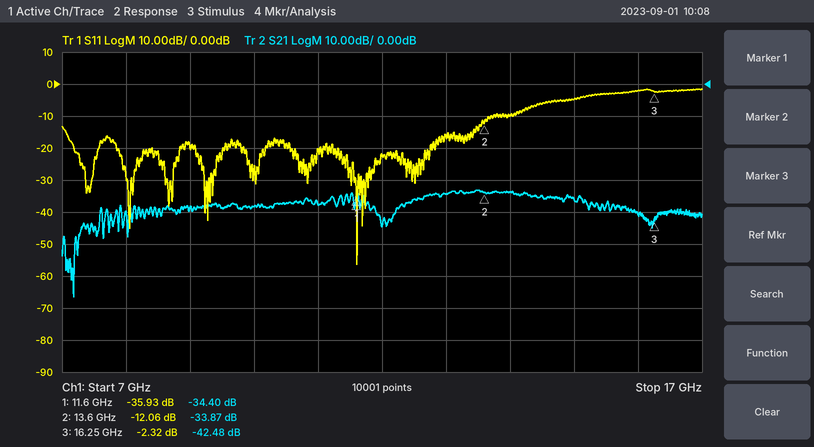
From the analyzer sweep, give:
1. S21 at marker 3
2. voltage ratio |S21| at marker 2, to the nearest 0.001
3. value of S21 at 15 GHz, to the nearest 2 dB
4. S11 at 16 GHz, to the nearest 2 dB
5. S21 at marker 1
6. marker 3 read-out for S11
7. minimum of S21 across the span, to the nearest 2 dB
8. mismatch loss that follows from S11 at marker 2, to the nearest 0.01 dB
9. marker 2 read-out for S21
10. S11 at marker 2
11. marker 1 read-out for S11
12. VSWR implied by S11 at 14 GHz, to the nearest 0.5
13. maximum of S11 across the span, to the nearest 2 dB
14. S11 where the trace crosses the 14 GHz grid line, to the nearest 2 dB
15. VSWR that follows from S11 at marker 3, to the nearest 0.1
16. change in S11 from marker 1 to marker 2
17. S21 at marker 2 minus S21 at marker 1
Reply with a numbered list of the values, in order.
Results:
1. -42.48 dB
2. 0.020
3. -36 dB
4. -2 dB
5. -34.40 dB
6. -2.32 dB
7. -66 dB
8. 0.28 dB
9. -33.87 dB
10. -12.06 dB
11. -35.93 dB
12. 2.0
13. -2 dB
14. -10 dB
15. 7.5
16. 23.87 dB
17. 0.53 dB
